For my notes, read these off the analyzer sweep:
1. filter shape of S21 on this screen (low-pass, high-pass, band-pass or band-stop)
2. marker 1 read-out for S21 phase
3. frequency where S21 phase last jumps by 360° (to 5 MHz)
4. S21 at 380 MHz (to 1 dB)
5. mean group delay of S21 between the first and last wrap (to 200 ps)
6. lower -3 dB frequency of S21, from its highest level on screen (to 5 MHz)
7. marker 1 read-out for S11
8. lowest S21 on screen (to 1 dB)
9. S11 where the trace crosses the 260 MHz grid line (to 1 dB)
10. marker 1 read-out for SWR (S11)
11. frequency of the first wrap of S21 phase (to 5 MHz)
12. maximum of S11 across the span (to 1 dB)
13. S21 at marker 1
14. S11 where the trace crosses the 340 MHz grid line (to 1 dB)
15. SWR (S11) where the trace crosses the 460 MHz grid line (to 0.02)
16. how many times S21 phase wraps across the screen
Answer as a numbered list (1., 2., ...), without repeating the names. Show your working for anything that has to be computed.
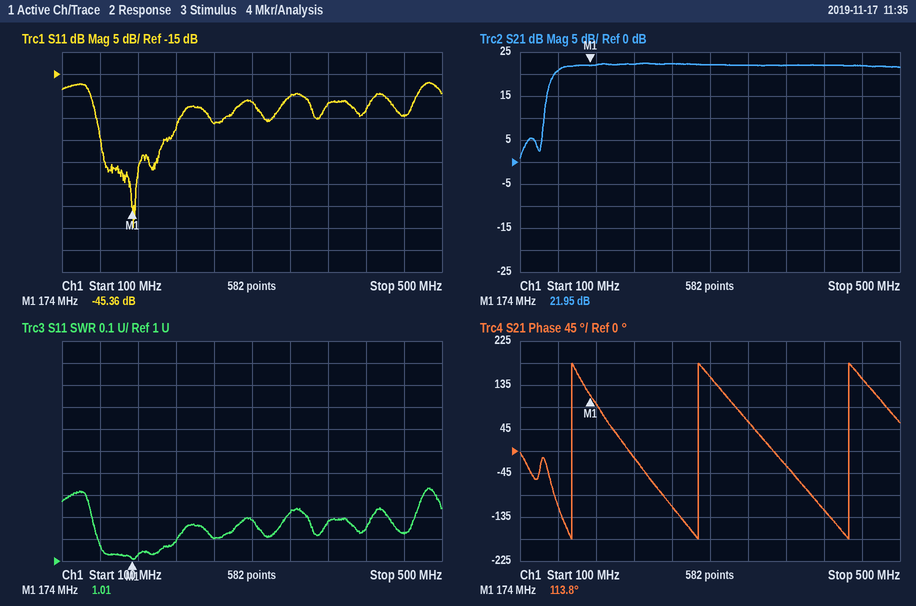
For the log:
1. high-pass
2. 113.8°
3. 445 MHz
4. 22 dB
5. 2 cycles / (445 MHz − 155 MHz) ≈ 6.90 ns, so 6.8 ns to the nearest 200 ps
6. 135 MHz
7. -45.36 dB
8. 1 dB
9. -26 dB
10. 1.01
11. 155 MHz
12. -17 dB
13. 21.95 dB
14. -20 dB
15. 1.12
16. 3
